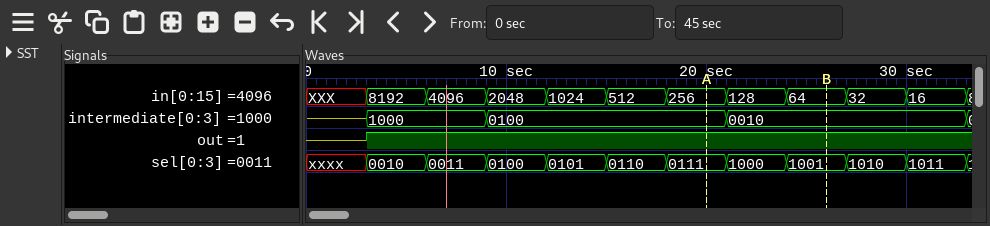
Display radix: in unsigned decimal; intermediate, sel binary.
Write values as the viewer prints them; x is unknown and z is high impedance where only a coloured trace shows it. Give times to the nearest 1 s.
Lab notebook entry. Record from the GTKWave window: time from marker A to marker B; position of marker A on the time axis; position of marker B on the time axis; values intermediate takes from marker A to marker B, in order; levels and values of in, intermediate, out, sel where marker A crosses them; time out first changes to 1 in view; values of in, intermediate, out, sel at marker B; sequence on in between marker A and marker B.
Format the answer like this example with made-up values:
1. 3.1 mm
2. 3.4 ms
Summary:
1. 6 s
2. 20 s
3. 26 s
4. 0100, 0010
5. in=256, intermediate=0100, out=1, sel=0111
6. 3 s
7. in=64, intermediate=0010, out=1, sel=1001
8. 256, 128, 64
